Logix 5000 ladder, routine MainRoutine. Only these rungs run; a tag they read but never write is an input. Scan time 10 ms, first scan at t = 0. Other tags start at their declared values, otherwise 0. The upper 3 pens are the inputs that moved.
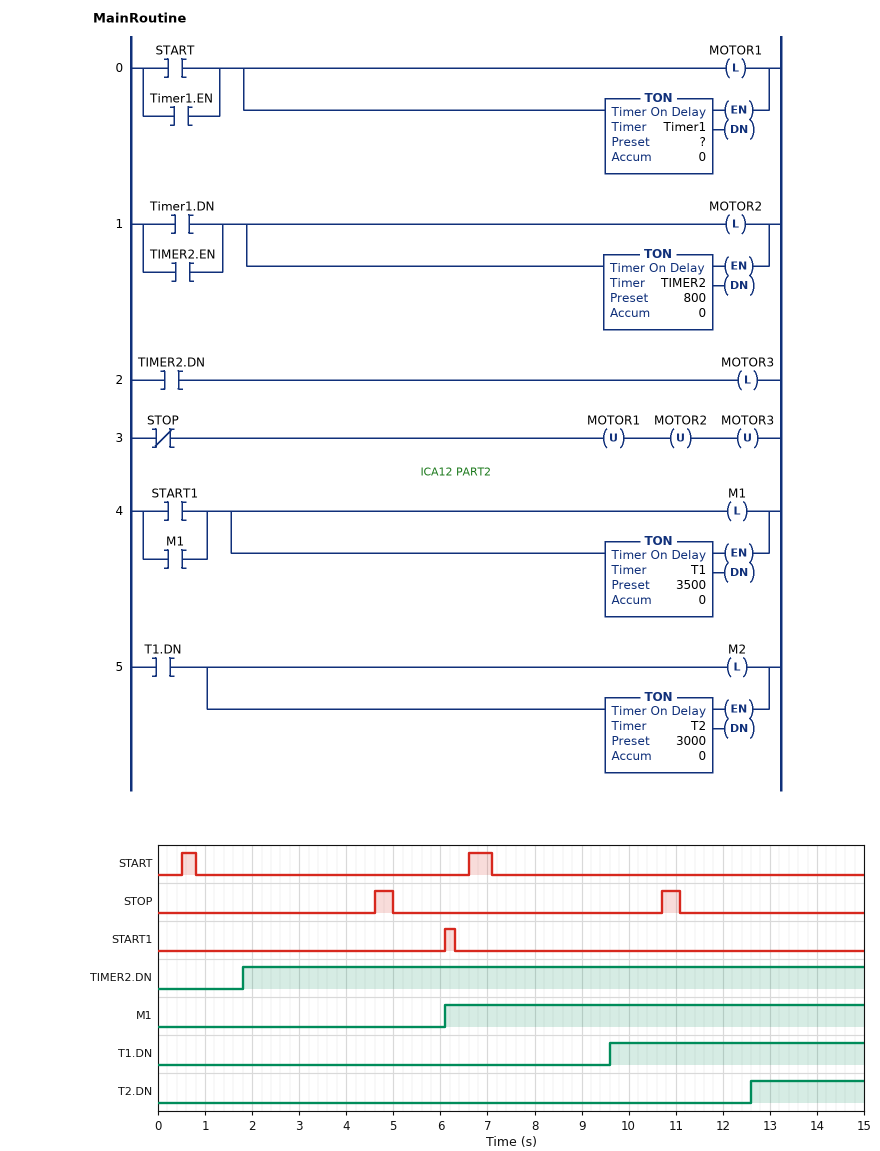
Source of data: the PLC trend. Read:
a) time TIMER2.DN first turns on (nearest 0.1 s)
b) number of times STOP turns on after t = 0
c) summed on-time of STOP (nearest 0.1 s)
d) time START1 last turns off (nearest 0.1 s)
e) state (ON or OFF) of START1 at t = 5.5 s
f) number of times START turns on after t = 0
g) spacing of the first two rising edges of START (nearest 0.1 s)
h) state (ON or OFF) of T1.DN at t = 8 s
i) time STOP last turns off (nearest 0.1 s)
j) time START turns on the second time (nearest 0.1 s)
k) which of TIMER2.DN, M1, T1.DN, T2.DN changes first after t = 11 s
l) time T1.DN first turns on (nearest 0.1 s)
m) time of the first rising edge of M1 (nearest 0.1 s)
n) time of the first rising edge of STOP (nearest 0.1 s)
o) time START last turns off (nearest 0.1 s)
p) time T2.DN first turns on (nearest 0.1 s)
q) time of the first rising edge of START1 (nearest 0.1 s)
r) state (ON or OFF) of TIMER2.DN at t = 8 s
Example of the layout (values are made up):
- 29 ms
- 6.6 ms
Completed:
- 1.8 s
- 2
- 0.8 s
- 6.3 s
- OFF
- 2
- 6.1 s
- OFF
- 11.1 s
- 6.6 s
- T2.DN
- 9.6 s
- 6.1 s
- 4.6 s
- 7.1 s
- 12.6 s
- 6.1 s
- ON
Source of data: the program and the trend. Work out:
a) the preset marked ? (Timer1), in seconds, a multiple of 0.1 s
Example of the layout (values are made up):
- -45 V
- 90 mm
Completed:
- 0.5 s
